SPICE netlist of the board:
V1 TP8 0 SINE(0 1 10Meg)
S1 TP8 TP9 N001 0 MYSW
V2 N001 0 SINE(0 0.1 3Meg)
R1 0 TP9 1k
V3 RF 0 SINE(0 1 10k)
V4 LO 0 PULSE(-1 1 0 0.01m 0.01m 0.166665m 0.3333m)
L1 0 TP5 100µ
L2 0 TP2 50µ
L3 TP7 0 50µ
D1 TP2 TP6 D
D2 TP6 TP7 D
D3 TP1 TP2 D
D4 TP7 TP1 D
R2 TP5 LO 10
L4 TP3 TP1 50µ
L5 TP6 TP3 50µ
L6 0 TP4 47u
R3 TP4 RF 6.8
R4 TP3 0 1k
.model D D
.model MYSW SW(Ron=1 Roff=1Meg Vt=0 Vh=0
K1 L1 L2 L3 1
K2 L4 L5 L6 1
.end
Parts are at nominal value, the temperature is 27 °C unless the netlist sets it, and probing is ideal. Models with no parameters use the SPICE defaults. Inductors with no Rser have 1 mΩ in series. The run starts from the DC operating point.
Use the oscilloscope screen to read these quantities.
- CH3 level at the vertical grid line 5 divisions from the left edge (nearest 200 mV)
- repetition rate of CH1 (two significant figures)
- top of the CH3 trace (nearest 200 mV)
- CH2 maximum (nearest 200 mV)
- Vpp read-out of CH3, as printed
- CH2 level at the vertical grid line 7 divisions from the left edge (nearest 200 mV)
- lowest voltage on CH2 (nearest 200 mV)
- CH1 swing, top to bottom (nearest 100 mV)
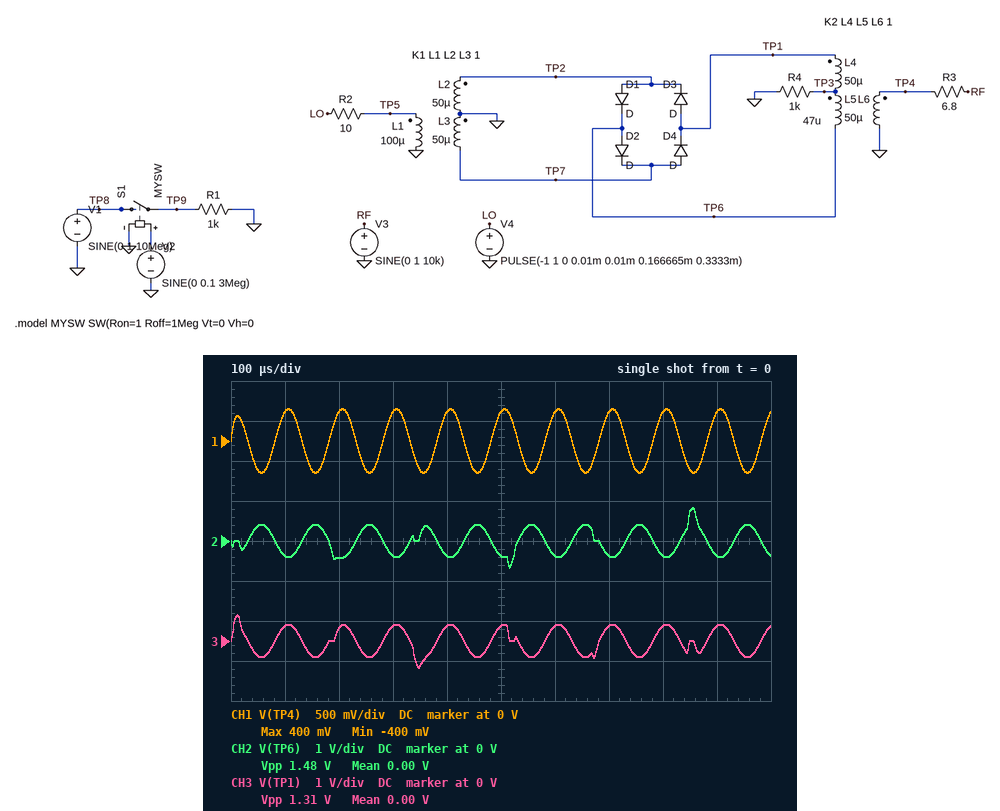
400 mV
10 kHz
600 mV
800 mV
1.31 V
-400 mV
-600 mV
800 mV
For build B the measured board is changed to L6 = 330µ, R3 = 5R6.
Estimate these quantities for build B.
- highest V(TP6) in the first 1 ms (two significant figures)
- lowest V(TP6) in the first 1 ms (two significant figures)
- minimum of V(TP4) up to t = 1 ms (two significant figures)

550 mV
-750 mV
-1.0 V
